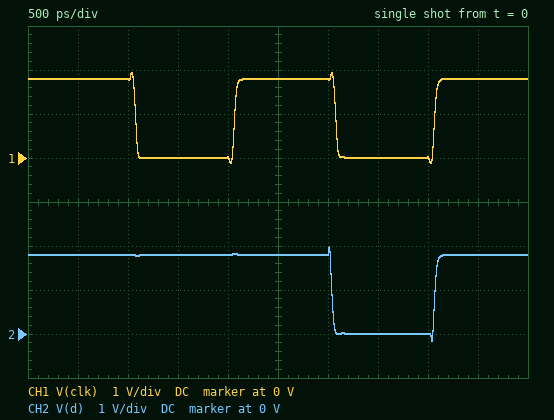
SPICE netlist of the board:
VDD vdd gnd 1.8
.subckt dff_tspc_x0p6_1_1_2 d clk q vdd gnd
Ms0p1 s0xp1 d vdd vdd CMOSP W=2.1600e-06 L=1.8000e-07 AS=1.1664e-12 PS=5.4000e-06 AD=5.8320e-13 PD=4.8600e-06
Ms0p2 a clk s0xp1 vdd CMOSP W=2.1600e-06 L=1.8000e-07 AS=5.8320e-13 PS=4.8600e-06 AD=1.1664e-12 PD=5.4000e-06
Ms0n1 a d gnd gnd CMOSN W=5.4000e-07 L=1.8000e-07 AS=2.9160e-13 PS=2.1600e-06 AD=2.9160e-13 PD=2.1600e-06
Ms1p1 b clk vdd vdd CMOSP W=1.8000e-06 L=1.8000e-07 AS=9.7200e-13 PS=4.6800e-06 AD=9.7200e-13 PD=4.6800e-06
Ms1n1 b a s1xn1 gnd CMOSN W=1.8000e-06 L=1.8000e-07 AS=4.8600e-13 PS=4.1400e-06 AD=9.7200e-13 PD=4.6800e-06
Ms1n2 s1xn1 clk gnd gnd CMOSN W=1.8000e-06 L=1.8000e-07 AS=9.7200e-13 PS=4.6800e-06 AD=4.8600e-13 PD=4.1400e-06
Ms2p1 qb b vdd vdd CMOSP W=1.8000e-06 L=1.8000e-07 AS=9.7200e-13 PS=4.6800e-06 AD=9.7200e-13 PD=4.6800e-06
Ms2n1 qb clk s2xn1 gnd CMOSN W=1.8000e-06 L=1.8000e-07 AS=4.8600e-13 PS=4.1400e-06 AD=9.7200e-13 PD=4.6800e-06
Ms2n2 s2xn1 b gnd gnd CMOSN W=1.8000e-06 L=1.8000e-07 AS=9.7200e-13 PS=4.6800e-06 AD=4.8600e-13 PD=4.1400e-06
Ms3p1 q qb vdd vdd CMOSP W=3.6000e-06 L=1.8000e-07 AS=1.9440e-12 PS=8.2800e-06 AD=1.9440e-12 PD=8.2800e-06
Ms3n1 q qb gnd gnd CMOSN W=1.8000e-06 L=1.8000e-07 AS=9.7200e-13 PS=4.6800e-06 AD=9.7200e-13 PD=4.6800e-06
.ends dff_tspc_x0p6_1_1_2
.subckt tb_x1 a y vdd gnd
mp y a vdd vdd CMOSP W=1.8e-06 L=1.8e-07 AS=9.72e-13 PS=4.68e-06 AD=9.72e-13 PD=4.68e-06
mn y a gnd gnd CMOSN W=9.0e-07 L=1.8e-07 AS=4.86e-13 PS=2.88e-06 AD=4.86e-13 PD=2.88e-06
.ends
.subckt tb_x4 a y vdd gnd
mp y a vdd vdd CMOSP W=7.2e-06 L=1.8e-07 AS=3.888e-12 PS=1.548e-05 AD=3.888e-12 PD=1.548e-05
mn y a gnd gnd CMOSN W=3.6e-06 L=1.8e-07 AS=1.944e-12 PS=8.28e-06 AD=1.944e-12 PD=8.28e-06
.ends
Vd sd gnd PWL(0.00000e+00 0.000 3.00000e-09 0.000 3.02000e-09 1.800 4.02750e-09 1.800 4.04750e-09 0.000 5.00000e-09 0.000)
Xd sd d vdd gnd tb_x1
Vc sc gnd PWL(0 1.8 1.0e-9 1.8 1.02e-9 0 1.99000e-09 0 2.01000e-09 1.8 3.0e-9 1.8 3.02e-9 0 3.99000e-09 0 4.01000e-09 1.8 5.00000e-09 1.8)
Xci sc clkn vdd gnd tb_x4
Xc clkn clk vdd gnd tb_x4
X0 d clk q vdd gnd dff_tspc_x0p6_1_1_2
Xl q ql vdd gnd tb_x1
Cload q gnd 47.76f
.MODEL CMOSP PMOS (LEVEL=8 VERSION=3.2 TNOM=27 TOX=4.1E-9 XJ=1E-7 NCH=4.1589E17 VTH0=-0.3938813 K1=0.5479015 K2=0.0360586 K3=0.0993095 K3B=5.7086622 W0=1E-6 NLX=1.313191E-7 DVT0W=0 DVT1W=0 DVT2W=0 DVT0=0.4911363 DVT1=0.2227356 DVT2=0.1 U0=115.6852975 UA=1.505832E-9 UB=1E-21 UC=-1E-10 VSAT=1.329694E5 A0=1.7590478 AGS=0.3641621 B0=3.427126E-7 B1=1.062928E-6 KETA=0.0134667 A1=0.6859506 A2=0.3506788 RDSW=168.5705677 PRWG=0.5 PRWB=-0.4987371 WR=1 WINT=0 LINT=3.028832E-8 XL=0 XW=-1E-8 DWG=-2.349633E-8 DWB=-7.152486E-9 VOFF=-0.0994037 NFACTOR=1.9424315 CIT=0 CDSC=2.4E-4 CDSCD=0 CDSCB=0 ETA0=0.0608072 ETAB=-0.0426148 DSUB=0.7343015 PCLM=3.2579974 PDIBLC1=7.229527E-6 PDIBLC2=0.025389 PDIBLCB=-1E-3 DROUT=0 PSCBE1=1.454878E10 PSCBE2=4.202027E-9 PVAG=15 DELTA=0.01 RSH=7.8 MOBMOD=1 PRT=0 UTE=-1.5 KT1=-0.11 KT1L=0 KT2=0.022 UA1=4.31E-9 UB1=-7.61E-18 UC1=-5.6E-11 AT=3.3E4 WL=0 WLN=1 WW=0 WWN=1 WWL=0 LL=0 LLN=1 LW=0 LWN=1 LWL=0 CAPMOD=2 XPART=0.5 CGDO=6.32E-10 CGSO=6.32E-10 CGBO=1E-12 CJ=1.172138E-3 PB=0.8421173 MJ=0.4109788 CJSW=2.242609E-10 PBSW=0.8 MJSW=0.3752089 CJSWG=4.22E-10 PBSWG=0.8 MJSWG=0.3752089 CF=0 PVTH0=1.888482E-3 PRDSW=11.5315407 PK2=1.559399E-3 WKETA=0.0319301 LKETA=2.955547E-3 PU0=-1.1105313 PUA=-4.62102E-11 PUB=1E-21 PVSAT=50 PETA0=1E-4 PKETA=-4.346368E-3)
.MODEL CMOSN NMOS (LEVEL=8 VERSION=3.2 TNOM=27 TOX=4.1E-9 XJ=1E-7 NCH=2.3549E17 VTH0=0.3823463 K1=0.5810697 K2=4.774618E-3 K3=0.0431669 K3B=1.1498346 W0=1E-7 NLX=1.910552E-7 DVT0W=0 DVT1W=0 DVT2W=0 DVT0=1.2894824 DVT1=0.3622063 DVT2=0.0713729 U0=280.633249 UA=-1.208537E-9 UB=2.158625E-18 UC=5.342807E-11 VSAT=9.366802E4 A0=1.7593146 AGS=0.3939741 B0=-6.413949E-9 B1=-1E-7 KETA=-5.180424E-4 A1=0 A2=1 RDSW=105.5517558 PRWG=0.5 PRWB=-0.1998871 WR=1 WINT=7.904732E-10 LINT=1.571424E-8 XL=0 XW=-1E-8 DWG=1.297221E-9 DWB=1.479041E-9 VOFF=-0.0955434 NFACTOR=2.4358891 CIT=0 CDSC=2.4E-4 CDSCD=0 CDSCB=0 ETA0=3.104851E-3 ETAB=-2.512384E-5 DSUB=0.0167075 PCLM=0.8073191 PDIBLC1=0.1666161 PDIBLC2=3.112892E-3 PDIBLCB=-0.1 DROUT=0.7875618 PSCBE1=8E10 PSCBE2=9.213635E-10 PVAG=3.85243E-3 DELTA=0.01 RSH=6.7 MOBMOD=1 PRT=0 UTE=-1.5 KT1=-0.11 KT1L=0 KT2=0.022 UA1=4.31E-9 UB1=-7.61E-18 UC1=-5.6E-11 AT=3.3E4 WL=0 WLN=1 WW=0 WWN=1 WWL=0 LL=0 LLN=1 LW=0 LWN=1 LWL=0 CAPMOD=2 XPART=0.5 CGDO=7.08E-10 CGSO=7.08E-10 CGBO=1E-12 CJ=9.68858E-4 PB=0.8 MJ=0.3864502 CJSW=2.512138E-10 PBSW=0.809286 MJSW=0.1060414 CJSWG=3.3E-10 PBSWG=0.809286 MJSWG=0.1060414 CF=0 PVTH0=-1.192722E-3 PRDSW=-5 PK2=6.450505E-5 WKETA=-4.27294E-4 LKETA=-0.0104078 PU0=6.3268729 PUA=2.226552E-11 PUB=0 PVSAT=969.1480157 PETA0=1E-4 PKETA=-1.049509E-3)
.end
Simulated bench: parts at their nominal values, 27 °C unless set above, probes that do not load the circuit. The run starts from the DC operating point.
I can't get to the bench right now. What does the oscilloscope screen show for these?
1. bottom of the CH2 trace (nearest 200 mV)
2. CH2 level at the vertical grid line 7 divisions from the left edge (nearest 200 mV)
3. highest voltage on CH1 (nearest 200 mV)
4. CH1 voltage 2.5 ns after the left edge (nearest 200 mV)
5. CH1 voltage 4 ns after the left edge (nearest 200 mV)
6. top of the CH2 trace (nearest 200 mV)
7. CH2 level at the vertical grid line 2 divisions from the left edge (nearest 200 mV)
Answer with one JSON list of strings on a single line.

["-200 mV", "0 V", "2.0 V", "1.8 V", "0 V", "2.0 V", "1.8 V"]
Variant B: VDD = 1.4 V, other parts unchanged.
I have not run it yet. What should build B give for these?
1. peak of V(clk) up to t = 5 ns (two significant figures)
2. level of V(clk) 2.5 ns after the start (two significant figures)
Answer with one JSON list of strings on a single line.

["1.5 V", "1.4 V"]
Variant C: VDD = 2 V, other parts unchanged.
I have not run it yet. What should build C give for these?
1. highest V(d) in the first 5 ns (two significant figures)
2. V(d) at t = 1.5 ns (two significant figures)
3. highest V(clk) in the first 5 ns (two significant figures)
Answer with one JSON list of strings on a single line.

["2.2 V", "2.0 V", "2.1 V"]
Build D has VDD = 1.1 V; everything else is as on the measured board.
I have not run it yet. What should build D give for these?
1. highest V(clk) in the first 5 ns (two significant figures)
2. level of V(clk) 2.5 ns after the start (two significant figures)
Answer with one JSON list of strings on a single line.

["1.2 V", "1.1 V"]
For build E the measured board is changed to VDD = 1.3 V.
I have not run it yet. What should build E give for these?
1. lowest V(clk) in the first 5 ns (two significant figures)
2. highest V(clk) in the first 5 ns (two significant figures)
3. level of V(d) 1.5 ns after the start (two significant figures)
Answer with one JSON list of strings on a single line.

["-170 mV", "1.4 V", "1.3 V"]
